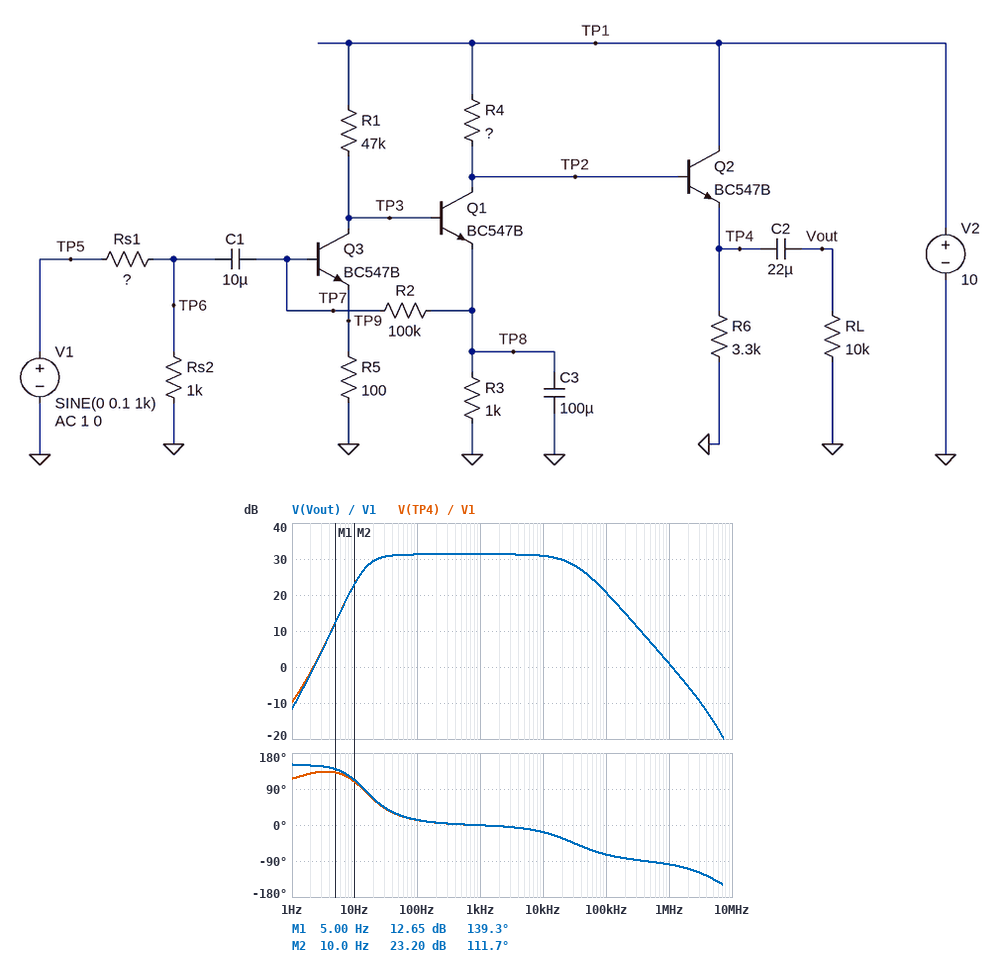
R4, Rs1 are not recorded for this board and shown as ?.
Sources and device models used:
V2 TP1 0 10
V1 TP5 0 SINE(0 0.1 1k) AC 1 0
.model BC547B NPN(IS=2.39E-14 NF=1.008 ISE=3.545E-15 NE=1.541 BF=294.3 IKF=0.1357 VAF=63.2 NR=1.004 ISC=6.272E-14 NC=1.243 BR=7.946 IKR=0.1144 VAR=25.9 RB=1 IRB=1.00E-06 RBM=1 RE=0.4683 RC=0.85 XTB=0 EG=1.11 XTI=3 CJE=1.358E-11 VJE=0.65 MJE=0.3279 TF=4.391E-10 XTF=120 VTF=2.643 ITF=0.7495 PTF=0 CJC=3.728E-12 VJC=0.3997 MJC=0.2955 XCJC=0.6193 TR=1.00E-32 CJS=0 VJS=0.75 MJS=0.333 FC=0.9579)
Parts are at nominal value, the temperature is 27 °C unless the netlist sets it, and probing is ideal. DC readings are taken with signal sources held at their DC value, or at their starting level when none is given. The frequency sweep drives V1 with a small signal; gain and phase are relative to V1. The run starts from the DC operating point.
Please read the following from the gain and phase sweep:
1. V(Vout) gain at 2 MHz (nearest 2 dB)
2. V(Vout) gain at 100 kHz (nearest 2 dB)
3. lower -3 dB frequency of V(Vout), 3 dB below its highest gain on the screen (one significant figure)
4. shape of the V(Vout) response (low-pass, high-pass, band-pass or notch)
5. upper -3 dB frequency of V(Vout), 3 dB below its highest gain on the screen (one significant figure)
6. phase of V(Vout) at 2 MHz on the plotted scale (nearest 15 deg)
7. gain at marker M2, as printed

-6 dB
20 dB
20 Hz
band-pass
30 kHz
-105 deg
23.20 dB
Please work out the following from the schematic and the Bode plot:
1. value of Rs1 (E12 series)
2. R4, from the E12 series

220 kΩ
10 kΩ
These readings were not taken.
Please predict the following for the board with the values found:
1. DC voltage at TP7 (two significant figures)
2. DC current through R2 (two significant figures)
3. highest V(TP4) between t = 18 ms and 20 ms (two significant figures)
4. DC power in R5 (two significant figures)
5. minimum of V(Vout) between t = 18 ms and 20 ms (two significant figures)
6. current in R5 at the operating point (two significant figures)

610 mV
640 nA
5.9 V
3.4 µW
-2.0 V
180 µA
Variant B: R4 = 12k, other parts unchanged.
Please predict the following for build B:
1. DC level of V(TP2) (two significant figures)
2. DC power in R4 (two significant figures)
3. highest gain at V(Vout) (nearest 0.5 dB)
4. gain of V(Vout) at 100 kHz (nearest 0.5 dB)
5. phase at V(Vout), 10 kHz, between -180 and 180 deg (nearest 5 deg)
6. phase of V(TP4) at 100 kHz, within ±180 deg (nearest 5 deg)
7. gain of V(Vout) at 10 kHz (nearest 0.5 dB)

1.9 V
5.5 mW
32.5 dB
19.0 dB
-25 deg
-80 deg
31.5 dB
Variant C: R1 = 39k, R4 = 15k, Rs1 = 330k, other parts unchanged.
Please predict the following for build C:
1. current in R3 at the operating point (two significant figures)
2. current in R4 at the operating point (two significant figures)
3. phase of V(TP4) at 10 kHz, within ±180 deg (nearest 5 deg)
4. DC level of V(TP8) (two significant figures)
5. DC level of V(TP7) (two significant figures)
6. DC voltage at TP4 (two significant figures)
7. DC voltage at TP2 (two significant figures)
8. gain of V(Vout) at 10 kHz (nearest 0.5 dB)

670 µA
620 µA
0 deg
670 mV
610 mV
150 mV
700 mV
-49.5 dB
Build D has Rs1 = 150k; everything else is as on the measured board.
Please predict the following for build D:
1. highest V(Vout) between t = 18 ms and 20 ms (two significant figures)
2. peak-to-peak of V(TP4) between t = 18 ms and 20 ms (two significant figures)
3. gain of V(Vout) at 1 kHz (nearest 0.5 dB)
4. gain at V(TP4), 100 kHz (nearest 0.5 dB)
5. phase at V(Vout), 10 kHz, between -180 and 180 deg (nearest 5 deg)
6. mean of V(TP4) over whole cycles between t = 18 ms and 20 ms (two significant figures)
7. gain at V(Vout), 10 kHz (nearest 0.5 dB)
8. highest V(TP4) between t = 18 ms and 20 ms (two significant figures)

4.1 V
6.1 V
34.5 dB
24.0 dB
-20 deg
2.8 V
34.0 dB
6.7 V
